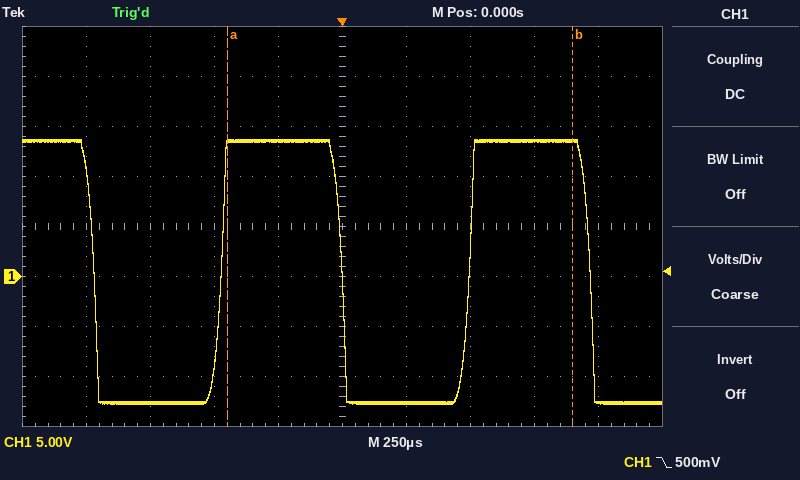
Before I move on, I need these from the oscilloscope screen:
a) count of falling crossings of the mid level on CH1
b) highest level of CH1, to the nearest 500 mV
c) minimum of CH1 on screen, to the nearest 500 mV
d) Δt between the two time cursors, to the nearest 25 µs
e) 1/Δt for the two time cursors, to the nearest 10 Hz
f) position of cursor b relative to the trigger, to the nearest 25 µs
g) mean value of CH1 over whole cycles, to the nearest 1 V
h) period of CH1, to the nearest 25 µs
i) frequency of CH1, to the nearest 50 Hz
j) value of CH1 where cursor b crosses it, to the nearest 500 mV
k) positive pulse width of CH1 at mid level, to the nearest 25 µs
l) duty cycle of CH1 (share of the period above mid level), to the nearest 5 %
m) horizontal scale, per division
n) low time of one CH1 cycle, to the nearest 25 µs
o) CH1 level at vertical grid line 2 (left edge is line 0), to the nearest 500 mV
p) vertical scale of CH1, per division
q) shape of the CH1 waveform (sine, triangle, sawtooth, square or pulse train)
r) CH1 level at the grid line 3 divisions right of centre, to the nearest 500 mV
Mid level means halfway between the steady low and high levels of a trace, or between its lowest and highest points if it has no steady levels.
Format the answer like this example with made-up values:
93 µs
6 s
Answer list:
3
13.5 V
-12.5 V
1.350 ms
740 Hz
+900 µs
0 V
975 µs
1.05 kHz
13.5 V
475 µs
50 %
250 µs
500 µs
-12.5 V
5 V
square
13.5 V
